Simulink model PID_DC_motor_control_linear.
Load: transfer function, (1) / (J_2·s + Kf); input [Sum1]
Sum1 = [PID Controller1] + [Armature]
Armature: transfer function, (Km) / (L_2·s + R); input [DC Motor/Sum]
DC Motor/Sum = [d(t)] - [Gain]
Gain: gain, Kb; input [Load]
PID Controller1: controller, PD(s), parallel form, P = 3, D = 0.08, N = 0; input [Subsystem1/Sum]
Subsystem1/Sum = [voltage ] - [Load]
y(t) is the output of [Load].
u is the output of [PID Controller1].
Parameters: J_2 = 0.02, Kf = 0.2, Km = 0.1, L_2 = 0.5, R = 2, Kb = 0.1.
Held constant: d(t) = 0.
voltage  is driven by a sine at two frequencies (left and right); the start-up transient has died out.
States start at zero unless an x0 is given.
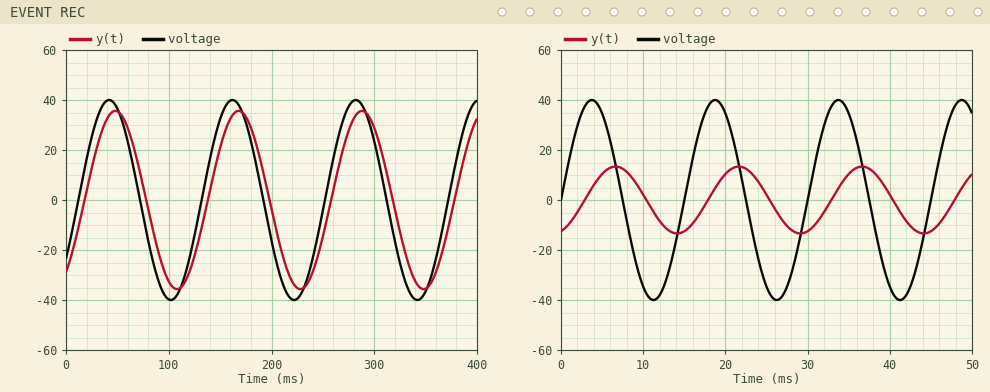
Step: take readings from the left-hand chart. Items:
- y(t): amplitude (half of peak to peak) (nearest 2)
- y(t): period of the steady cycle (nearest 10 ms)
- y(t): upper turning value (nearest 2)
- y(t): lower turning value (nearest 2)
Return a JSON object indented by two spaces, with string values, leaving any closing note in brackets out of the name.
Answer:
{
  "y(t): amplitude (half of peak to peak)": "36",
  "y(t): period of the steady cycle": "120 ms",
  "y(t): upper turning value": "36",
  "y(t): lower turning value": "-36"
}
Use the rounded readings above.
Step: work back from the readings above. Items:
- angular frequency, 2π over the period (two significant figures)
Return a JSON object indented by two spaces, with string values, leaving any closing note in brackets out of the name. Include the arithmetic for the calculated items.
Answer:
{
  "angular frequency, 2π over the period": "2π / 120 = 0.052 rad/ms"
}
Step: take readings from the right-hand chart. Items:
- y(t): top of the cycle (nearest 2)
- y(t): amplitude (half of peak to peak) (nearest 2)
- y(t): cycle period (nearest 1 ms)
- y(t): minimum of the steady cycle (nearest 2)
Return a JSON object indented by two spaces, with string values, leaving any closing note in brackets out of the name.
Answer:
{
  "y(t): top of the cycle": "14",
  "y(t): amplitude (half of peak to peak)": "14",
  "y(t): cycle period": "15 ms",
  "y(t): minimum of the steady cycle": "-14"
}
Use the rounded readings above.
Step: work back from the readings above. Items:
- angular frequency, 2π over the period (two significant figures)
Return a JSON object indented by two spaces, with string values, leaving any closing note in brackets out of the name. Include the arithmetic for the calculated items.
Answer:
{
  "angular frequency, 2π over the period": "2π / 15 = 0.42 rad/ms"
}
